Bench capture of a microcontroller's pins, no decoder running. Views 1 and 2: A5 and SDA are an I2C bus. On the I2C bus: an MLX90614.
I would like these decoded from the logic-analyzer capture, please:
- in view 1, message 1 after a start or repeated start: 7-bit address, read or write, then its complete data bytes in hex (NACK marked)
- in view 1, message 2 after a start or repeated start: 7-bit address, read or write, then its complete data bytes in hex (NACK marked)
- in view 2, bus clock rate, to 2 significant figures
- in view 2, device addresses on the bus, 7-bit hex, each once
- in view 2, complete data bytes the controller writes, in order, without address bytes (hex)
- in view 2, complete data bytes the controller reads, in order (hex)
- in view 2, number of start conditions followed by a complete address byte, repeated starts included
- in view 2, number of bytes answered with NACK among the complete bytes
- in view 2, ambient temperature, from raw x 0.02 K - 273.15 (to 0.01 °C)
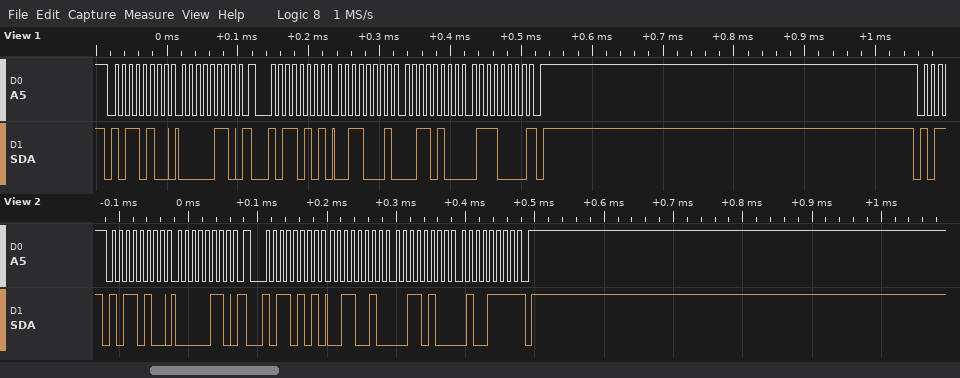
0x5A write: 06
0x5A read: 31 34 70 NACK
100 kHz
0x5A
06
32 34 4F
2
1
-5.91 °C
